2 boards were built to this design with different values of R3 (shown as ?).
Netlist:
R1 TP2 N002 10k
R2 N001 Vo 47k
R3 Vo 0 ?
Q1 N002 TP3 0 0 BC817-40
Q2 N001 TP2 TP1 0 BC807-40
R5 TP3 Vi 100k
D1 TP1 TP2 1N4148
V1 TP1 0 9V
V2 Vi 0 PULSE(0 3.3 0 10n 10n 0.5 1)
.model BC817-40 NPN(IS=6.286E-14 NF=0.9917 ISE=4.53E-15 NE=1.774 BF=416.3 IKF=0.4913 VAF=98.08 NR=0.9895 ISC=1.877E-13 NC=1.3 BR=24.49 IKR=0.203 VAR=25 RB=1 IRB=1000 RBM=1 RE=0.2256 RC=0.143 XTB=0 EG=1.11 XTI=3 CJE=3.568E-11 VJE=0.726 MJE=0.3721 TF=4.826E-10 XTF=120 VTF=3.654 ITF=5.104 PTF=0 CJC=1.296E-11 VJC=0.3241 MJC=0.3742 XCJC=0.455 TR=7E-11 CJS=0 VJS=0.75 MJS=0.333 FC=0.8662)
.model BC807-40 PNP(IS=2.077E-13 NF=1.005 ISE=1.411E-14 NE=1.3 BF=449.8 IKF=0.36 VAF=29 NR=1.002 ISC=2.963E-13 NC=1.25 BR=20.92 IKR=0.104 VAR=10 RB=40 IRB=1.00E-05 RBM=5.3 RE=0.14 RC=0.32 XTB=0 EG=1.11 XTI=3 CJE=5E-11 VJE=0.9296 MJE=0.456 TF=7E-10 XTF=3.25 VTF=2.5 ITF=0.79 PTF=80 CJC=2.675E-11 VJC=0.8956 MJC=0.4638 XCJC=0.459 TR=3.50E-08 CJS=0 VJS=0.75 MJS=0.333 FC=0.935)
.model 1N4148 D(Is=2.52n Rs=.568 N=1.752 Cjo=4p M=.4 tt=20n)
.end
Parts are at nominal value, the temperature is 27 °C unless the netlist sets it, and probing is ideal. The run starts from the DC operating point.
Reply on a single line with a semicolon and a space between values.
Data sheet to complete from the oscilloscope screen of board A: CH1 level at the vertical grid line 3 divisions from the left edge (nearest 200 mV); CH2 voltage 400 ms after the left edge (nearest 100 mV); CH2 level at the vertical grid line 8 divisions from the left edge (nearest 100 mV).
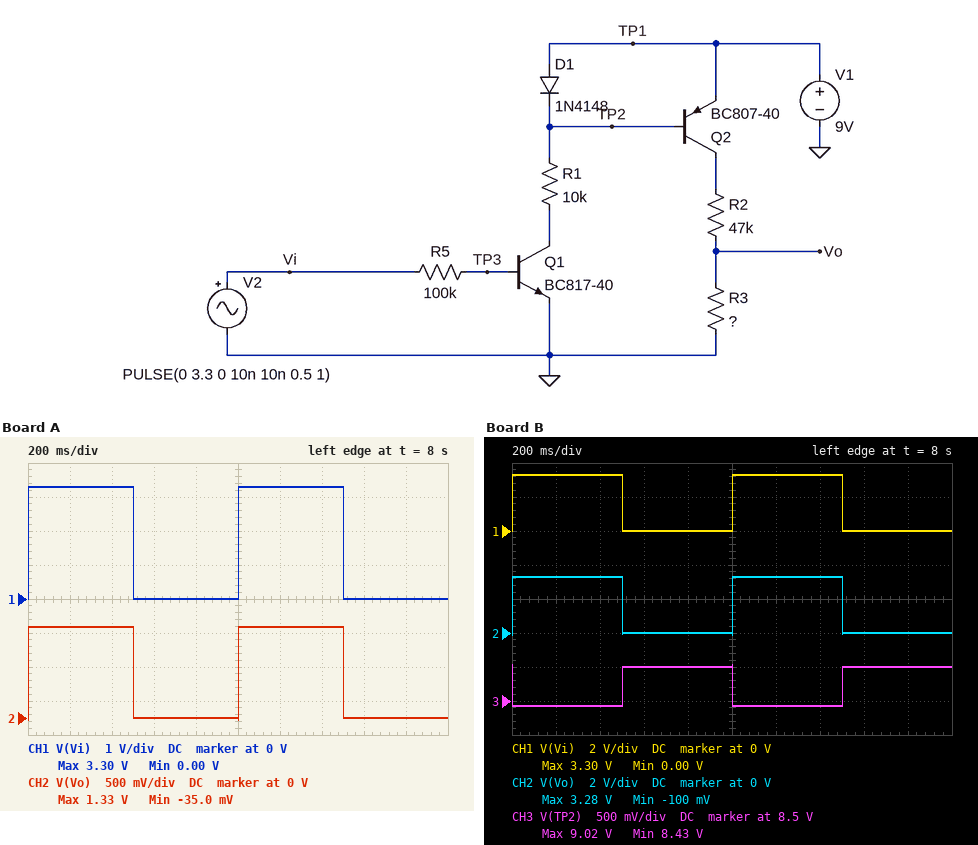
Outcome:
0 V; 1.3 V; 0 V
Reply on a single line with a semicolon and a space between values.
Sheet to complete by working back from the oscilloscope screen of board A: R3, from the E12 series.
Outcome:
8.2 kΩ
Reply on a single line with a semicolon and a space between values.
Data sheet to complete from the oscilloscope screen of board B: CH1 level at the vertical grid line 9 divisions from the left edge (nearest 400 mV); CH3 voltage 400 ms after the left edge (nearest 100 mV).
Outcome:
0 V; 8.4 V
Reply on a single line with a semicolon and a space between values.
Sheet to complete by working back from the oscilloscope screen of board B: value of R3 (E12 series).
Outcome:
27 kΩ
